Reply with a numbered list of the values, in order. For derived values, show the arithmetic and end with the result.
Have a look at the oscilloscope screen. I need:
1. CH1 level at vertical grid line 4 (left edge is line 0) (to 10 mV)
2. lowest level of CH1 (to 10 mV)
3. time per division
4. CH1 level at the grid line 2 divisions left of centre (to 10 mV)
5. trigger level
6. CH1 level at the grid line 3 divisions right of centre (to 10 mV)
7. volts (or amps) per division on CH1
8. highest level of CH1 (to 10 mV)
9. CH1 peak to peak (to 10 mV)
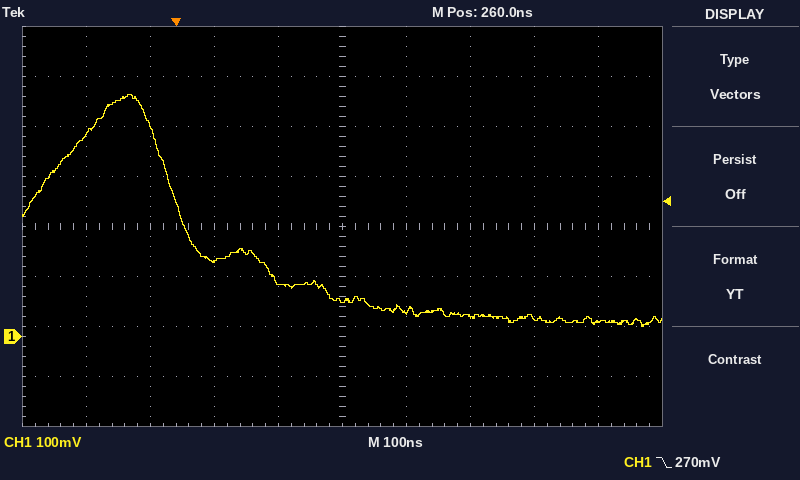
1. 110 mV
2. 20 mV
3. 100 ns
4. 150 mV
5. 270 mV
6. 40 mV
7. 100 mV
8. 480 mV
9. 480 mV − (20 mV) = 460 mV
